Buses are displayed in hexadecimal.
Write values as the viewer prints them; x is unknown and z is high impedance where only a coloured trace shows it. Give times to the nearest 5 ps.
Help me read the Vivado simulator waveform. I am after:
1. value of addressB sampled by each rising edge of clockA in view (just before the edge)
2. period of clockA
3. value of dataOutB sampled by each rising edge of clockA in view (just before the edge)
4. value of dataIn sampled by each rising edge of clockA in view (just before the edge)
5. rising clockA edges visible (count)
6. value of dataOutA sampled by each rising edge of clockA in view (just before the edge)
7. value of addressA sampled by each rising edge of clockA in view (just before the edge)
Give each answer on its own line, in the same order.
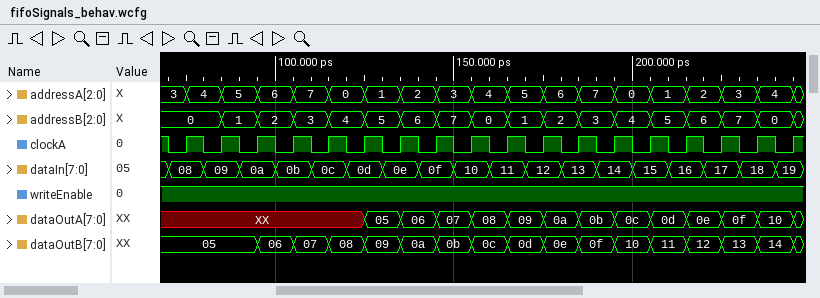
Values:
0, 0, 1, 2, 3, 4, 5, 6, 7, 0, 1, 2, 3, 4, 5, 6, 7, 0
10 ps
05, 05, 05, 06, 07, 08, 09, 0a, 0b, 0c, 0d, 0e, 0f, 10, 11, 12, 13, 14
08, 09, 0a, 0b, 0c, 0d, 0e, 0f, 10, 11, 12, 13, 14, 15, 16, 17, 18, 19
18
XX, XX, XX, XX, XX, XX, 05, 06, 07, 08, 09, 0a, 0b, 0c, 0d, 0e, 0f, 10
3, 4, 5, 6, 7, 0, 1, 2, 3, 4, 5, 6, 7, 0, 1, 2, 3, 4
